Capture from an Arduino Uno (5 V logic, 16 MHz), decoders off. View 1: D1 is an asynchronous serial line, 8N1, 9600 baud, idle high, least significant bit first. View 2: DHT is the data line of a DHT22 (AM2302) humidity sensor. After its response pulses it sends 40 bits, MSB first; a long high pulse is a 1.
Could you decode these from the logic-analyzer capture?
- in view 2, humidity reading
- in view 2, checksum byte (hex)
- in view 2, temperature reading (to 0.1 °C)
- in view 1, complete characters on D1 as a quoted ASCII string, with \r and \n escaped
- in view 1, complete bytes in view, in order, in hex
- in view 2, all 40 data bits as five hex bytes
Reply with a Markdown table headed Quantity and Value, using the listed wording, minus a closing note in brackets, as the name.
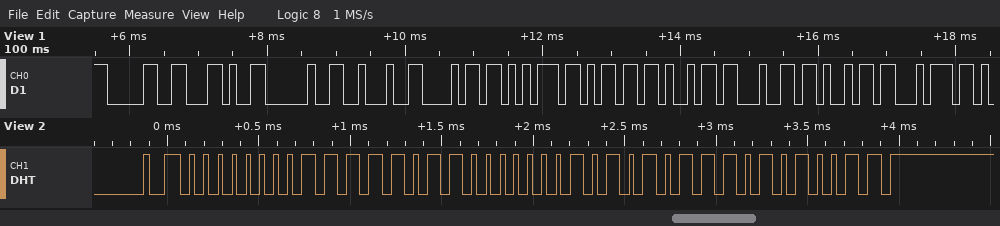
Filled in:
| Quantity | Value |
|---|---|
| in view 2, humidity reading | 25.1 % |
| in view 2, checksum byte | 0x53 |
| in view 2, temperature reading | 34.3 °C |
| in view 1, complete characters on D1 as a quoted ASCII string, with \r and \n escaped | "0, \"humidit" |
| in view 1, complete bytes in view, in order, in hex | 30 2C 20 22 68 75 6D 69 64 69 74 |
| in view 2, all 40 data bits as five hex bytes | 00 FB 01 57 53 |
